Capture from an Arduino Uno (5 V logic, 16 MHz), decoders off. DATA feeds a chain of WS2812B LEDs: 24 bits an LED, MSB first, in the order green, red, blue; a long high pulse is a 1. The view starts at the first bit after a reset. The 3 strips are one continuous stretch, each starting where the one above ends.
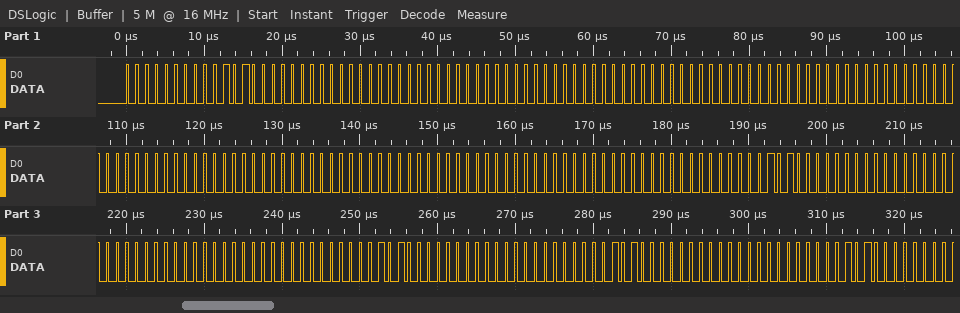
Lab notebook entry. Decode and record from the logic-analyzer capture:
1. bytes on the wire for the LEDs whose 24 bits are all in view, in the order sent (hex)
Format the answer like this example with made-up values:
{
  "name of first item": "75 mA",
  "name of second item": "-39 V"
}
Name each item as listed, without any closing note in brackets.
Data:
{
  "bytes on the wire for the LEDs whose 24 bits are all in view, in the order sent": "00 28 00 00 00 00 00 00 00 00 00 00 00 00 00 00 00 00 00 28 00 00 00 00 00 28 00 00 28 00"
}
